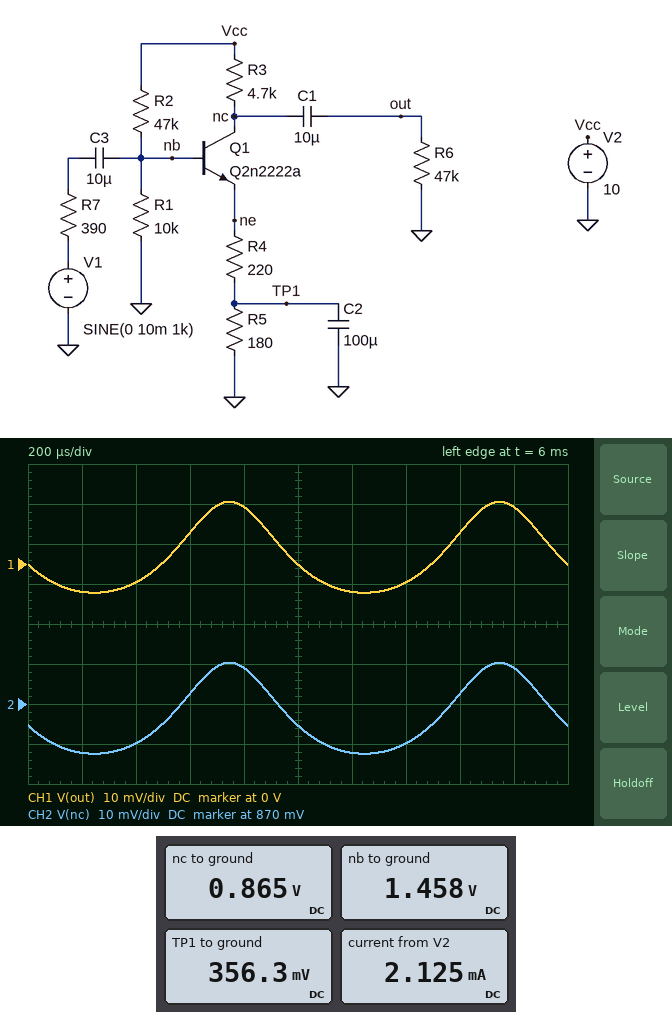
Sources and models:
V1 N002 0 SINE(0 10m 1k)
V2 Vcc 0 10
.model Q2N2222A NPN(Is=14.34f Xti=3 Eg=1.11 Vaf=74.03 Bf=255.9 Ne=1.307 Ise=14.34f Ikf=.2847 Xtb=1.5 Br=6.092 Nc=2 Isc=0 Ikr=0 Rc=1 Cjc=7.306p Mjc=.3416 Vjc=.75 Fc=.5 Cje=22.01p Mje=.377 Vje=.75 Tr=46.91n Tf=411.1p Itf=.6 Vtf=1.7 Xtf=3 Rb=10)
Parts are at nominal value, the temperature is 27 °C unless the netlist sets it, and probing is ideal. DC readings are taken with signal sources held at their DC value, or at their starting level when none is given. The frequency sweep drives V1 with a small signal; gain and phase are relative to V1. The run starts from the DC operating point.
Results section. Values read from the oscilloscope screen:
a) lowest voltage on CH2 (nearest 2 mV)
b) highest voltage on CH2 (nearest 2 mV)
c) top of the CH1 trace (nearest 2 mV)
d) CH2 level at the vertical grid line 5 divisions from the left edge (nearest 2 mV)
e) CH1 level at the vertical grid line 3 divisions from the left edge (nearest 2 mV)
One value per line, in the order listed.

858 mV
880 mV
16 mV
864 mV
8 mV
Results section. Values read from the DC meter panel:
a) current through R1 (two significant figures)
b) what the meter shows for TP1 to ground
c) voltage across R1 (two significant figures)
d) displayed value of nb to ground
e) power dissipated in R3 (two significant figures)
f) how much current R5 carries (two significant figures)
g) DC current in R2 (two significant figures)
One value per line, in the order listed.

150 µA
356.3 mV
1.5 V
1.458 V
18 mW
2.0 mA
180 µA
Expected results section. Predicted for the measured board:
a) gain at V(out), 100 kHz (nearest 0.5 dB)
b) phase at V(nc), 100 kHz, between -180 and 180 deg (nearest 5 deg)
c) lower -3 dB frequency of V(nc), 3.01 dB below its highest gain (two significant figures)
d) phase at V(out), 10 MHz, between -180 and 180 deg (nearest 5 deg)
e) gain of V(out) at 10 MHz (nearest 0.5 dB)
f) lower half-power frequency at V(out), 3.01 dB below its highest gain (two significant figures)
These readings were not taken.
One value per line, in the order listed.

0 dB
170 deg
26 Hz
15 deg
-9.0 dB
26 Hz
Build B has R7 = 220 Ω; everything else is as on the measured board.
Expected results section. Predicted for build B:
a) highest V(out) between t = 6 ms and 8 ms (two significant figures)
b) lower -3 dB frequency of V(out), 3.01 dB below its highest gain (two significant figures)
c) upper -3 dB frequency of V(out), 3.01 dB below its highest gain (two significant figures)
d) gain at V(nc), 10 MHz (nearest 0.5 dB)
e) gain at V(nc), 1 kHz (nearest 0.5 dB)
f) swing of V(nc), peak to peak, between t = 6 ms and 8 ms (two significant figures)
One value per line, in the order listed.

24 mV
33 Hz
820 kHz
-6.0 dB
2.0 dB
33 mV
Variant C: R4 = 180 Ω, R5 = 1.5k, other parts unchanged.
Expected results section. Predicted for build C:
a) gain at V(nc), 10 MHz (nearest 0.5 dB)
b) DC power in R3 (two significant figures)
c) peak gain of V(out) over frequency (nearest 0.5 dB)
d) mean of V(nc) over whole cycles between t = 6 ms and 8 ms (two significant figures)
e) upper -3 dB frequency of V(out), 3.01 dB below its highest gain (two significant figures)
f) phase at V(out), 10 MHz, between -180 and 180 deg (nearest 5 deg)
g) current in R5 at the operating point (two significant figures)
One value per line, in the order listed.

15.5 dB
1.9 mW
25.0 dB
7.0 V
3.5 MHz
100 deg
650 µA
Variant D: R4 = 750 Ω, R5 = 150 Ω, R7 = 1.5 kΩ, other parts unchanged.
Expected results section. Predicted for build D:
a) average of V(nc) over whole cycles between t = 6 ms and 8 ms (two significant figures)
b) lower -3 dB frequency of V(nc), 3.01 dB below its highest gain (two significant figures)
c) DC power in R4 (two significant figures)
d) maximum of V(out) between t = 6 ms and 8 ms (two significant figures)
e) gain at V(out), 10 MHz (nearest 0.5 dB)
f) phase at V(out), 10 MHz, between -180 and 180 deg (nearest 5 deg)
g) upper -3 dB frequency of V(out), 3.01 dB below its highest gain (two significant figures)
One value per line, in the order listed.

4.6 V
2.6 Hz
1.0 mW
46 mV
2.5 dB
90 deg
2.9 MHz
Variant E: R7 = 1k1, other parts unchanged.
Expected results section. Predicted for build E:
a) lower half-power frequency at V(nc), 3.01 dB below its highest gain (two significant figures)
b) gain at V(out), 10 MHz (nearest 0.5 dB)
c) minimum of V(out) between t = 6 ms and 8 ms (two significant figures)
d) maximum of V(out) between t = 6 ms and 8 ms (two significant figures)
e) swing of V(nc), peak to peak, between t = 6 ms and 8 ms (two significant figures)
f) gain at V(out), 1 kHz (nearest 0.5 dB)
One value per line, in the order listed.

15 Hz
-15.5 dB
-4.2 mV
6.2 mV
10 mV
-6.0 dB
